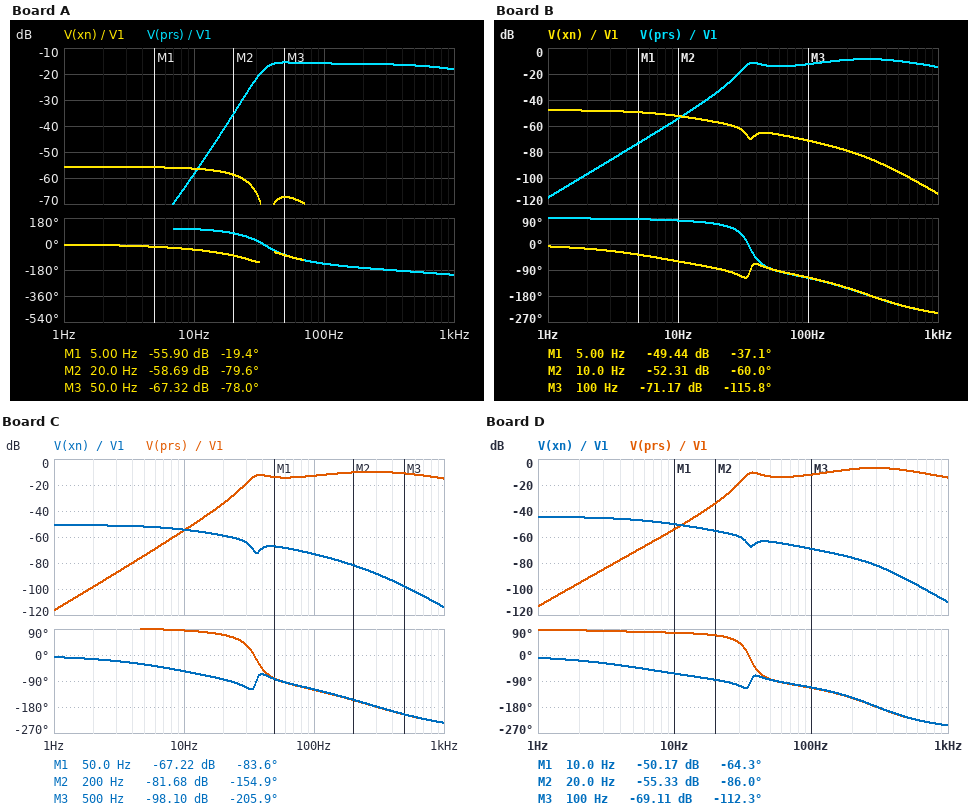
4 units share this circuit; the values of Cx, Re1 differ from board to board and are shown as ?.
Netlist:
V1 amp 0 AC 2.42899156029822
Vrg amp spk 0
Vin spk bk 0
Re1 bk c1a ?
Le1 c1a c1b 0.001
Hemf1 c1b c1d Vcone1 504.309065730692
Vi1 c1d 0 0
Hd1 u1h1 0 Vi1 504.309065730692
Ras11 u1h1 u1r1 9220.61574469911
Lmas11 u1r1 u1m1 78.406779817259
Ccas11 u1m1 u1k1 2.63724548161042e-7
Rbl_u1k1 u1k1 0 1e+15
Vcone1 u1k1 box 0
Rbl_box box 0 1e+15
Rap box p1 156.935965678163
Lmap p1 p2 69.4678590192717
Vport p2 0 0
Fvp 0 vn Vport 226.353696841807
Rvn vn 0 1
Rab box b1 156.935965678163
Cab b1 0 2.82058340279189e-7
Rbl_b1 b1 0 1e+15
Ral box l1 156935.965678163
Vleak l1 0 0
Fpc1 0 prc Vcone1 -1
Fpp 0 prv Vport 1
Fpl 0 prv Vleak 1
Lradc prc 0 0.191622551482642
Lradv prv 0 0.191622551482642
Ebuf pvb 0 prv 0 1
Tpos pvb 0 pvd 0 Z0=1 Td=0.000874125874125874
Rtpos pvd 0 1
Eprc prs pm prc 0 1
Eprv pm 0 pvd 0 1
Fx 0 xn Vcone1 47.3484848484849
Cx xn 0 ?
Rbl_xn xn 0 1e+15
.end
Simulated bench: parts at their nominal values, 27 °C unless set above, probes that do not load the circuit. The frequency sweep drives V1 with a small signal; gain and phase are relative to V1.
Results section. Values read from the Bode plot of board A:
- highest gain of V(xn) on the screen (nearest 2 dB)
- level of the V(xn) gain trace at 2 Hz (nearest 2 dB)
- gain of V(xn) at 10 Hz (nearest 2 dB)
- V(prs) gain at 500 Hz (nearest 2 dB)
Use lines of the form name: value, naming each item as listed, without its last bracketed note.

highest gain of V(xn) on the screen: -56 dB
level of the V(xn) gain trace at 2 Hz: -56 dB
gain of V(xn) at 10 Hz: -56 dB
V(prs) gain at 500 Hz: -16 dB
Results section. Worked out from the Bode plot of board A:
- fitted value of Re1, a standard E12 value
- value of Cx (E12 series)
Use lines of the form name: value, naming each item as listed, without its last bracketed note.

fitted value of Re1, a standard E12 value: 8.2 Ω
value of Cx: 470 mF
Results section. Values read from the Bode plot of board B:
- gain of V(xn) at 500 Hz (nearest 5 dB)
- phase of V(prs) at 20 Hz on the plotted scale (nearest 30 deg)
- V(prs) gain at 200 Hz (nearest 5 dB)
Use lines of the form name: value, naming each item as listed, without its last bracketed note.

gain of V(xn) at 500 Hz: -95 dB
phase of V(prs) at 20 Hz on the plotted scale: 60 deg
V(prs) gain at 200 Hz: -10 dB
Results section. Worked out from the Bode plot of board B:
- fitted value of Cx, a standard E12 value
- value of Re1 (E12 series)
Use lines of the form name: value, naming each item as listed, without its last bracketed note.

fitted value of Cx, a standard E12 value: 470 mF
value of Re1: 3.3 Ω
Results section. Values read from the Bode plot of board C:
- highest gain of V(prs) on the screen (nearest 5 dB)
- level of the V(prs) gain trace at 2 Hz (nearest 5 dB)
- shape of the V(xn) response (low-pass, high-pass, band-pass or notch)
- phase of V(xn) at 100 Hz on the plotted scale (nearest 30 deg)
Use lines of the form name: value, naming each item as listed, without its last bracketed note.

highest gain of V(prs) on the screen: -10 dB
level of the V(prs) gain trace at 2 Hz: -100 dB
shape of the V(xn) response: low-pass
phase of V(xn) at 100 Hz on the plotted scale: -120 deg
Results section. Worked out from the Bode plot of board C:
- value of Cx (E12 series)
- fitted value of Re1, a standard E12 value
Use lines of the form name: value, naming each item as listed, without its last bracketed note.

value of Cx: 560 mF
fitted value of Re1, a standard E12 value: 3.9 Ω
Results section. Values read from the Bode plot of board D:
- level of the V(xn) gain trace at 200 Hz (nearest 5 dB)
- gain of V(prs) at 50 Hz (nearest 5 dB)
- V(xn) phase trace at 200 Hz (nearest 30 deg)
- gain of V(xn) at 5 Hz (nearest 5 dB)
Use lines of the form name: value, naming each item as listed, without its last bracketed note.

level of the V(xn) gain trace at 200 Hz: -75 dB
gain of V(prs) at 50 Hz: -15 dB
V(xn) phase trace at 200 Hz: -150 deg
gain of V(xn) at 5 Hz: -45 dB
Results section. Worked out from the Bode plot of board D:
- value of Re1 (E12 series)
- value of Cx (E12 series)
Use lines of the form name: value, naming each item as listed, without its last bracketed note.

value of Re1: 2.7 Ω
value of Cx: 390 mF
